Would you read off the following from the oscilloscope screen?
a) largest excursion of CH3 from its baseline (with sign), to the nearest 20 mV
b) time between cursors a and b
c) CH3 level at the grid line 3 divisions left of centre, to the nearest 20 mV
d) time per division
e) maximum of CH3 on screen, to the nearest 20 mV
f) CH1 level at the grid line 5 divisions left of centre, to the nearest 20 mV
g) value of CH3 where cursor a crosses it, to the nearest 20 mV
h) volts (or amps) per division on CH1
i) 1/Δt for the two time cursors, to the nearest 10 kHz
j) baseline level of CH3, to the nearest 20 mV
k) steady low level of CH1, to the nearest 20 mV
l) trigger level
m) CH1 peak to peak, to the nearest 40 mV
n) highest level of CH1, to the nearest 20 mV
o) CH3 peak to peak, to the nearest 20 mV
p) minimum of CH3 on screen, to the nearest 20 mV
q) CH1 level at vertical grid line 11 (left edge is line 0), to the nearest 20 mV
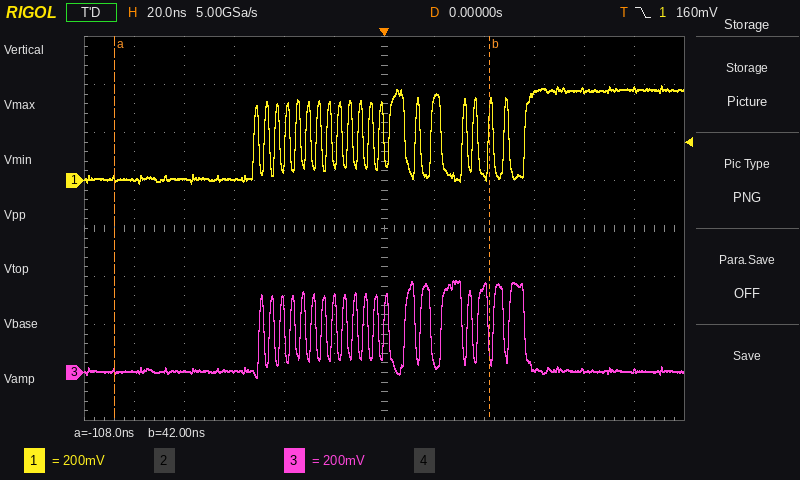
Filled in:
+380 mV
150 ns
0 mV
20 ns
380 mV
0 mV
0 mV
200 mV
6.67 MHz
0 mV
0 mV
160 mV
400 mV
400 mV
400 mV
-20 mV
380 mV
